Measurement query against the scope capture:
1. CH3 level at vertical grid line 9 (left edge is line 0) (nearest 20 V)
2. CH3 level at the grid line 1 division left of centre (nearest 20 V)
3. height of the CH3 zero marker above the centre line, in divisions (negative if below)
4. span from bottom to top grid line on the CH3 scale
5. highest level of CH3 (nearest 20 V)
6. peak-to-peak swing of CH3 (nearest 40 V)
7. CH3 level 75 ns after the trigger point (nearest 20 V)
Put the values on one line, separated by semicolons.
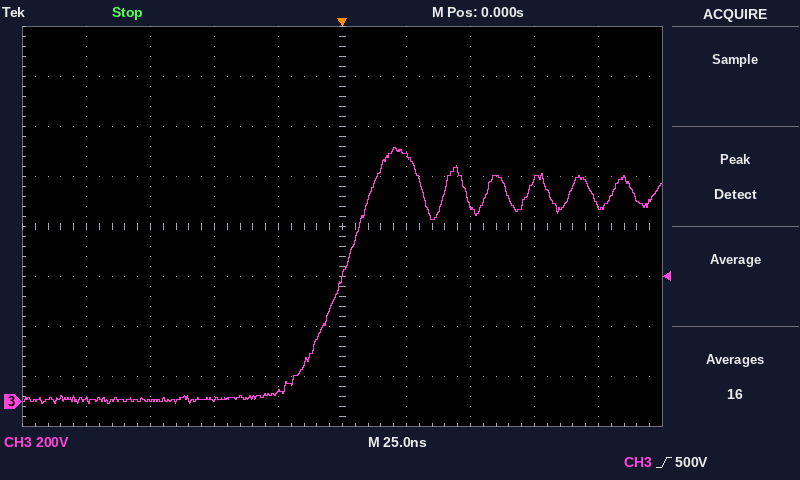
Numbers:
780 V; 40 V; -3.5 div; 1.6 kV; 1.02 kV; 1.04 kV; 880 V
